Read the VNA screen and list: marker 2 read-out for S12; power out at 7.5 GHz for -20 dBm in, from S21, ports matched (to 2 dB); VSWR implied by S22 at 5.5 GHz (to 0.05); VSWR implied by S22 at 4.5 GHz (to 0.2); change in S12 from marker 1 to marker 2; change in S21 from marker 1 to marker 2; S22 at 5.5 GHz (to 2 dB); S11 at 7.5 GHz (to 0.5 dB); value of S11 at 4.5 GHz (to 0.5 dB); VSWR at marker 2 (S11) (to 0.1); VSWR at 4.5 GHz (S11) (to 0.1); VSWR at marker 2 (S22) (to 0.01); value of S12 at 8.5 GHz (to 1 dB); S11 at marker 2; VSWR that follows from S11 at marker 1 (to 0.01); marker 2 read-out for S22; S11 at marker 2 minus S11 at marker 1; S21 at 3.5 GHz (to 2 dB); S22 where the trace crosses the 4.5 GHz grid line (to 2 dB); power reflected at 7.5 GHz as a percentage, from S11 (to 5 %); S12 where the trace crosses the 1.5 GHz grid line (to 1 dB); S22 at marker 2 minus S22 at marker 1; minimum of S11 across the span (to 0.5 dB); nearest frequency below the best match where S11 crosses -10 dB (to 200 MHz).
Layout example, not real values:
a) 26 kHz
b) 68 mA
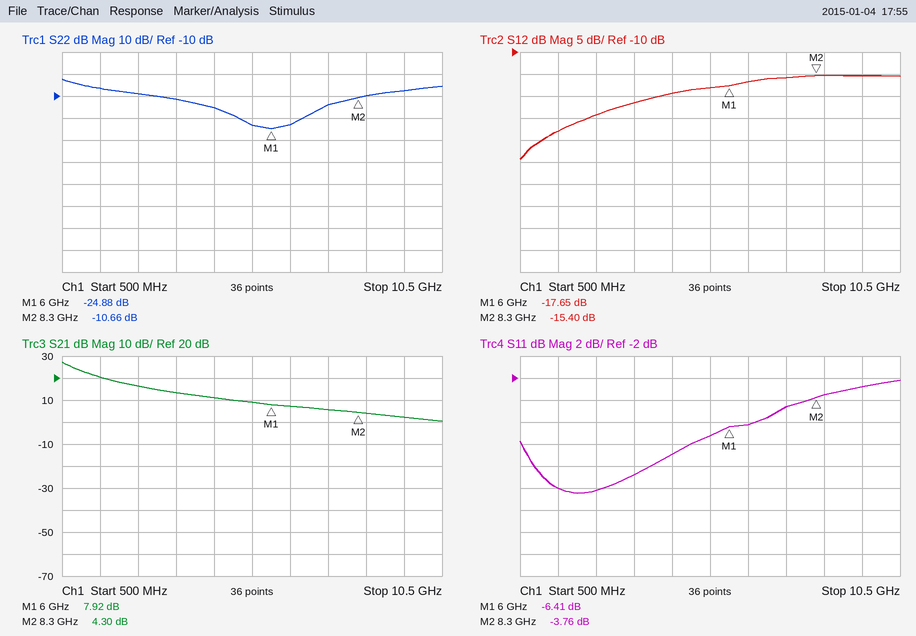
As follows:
a) -15.40 dB
b) -14 dBm
c) 1.15
d) 1.4
e) 2.25 dB
f) -3.62 dB
g) -24 dB
h) -4.5 dB
i) -9.0 dB
j) 4.7
k) 2.1
l) 1.83
m) -15 dB
n) -3.76 dB
o) 2.83
p) -10.66 dB
q) 2.65 dB
r) 14 dB
s) -16 dB
t) 35 %
u) -28 dB
v) 14.22 dB
w) -12.5 dB
x) 800 MHz
